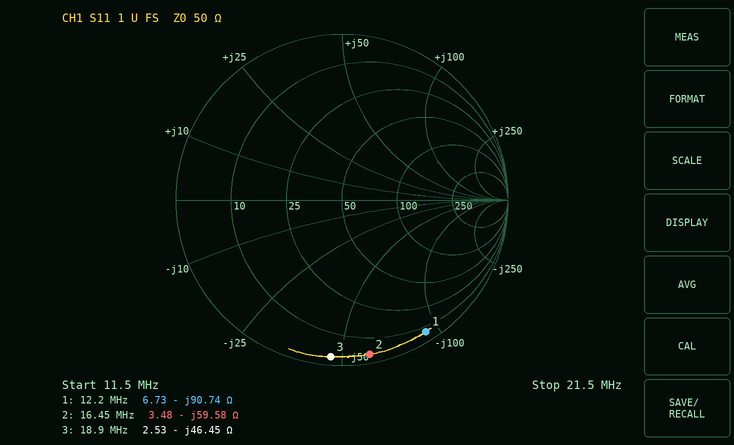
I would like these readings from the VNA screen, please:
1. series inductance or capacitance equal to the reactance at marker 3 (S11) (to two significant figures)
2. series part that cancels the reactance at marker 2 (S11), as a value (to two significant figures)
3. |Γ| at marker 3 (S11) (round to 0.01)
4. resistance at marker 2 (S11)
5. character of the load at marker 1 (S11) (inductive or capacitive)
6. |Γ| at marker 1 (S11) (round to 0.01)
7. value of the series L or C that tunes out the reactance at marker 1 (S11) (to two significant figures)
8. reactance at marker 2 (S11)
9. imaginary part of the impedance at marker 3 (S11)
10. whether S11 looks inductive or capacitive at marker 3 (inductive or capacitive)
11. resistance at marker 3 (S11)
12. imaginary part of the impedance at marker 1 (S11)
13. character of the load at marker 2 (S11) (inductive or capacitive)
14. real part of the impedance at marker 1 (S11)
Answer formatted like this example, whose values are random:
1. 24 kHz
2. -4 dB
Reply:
1. 180 pF
2. 580 nH
3. 0.95
4. 3.48 Ω
5. capacitive
6. 0.94
7. 1.2 µH
8. -59.58 Ω
9. -46.45 Ω
10. capacitive
11. 2.53 Ω
12. -90.74 Ω
13. capacitive
14. 6.73 Ω
